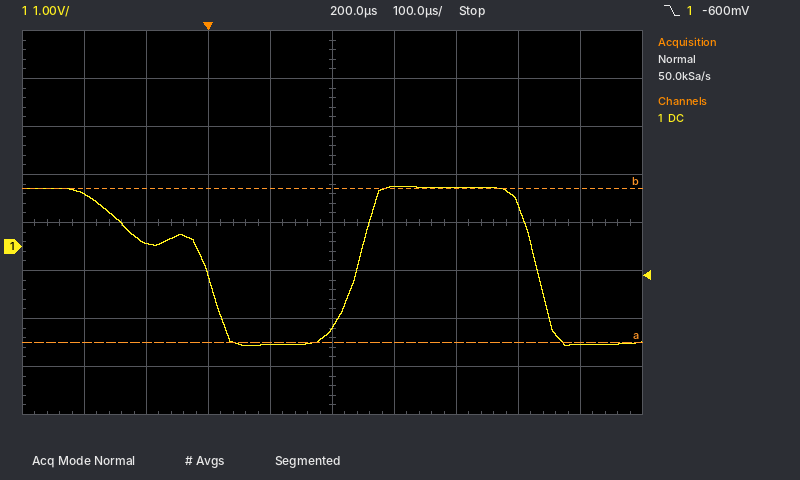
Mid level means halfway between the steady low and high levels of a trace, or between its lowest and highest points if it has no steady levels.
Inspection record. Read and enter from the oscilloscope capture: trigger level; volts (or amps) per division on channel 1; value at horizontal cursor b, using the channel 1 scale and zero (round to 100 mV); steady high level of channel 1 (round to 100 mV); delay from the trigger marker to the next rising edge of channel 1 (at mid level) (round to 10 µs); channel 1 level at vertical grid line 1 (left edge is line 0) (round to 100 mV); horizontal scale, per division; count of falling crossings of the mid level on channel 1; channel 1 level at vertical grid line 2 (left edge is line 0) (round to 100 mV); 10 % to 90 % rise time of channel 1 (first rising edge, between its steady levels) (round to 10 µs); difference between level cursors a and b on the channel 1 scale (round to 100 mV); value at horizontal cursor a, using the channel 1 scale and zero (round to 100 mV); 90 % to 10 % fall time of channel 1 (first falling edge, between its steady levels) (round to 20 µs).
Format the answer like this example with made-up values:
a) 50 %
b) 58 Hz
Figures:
a) -600 mV
b) 1 V
c) 1.2 V
d) 1.2 V
e) 240 µs
f) 1.1 V
g) 100 µs
h) 2
i) 100 mV
j) 70 µs
k) 3.2 V
l) -2.0 V
m) 200 µs
